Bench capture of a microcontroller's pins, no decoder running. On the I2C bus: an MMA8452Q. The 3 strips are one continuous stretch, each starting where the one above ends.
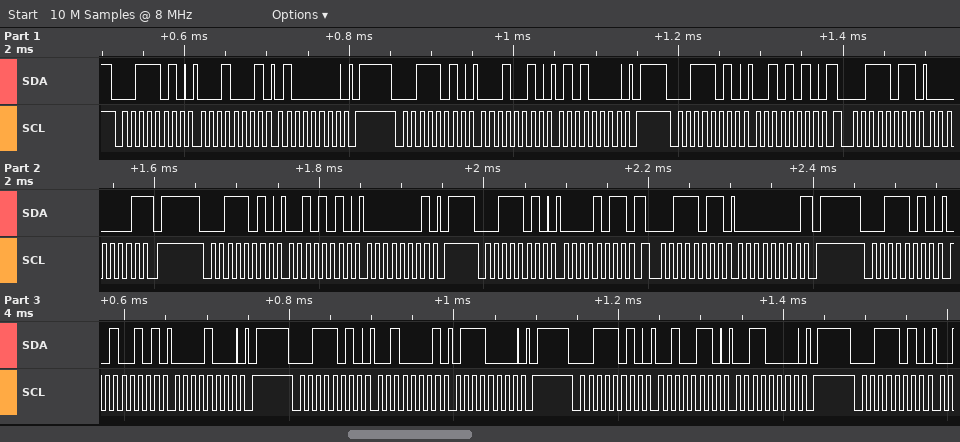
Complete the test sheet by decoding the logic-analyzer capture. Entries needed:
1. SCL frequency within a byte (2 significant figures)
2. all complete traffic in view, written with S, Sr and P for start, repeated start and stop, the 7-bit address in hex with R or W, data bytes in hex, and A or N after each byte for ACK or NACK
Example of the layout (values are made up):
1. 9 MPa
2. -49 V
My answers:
1. 100 kHz
2. S 1DW A 11 A 40 A P S 1DW A 12 A 50 A P S 1DW A 2A A Sr 1DR A 01 N P S 1DW A 2A A 01 A P S 1DW A 0B A Sr 1DR A 00 N P S 1DW A 25 A 08 A P S 1DW A 21 A 70 A P S 1DW A 26 A 30 A P S 1DW A
